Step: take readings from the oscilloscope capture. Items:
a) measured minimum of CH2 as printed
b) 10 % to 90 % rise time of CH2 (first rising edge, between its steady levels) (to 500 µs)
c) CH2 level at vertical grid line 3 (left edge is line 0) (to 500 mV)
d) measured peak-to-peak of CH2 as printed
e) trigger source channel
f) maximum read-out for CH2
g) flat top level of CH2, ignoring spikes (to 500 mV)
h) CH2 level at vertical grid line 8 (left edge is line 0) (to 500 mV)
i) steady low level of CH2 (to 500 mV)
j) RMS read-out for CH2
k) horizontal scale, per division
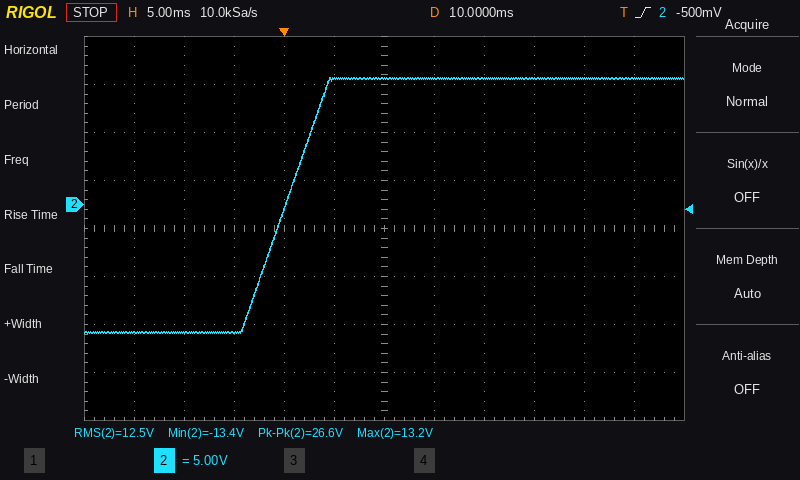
-13.4 V
7.0 ms
-13.5 V
26.6 V
CH2
13.2 V
13.0 V
13.0 V
-13.5 V
12.5 V
5 ms
